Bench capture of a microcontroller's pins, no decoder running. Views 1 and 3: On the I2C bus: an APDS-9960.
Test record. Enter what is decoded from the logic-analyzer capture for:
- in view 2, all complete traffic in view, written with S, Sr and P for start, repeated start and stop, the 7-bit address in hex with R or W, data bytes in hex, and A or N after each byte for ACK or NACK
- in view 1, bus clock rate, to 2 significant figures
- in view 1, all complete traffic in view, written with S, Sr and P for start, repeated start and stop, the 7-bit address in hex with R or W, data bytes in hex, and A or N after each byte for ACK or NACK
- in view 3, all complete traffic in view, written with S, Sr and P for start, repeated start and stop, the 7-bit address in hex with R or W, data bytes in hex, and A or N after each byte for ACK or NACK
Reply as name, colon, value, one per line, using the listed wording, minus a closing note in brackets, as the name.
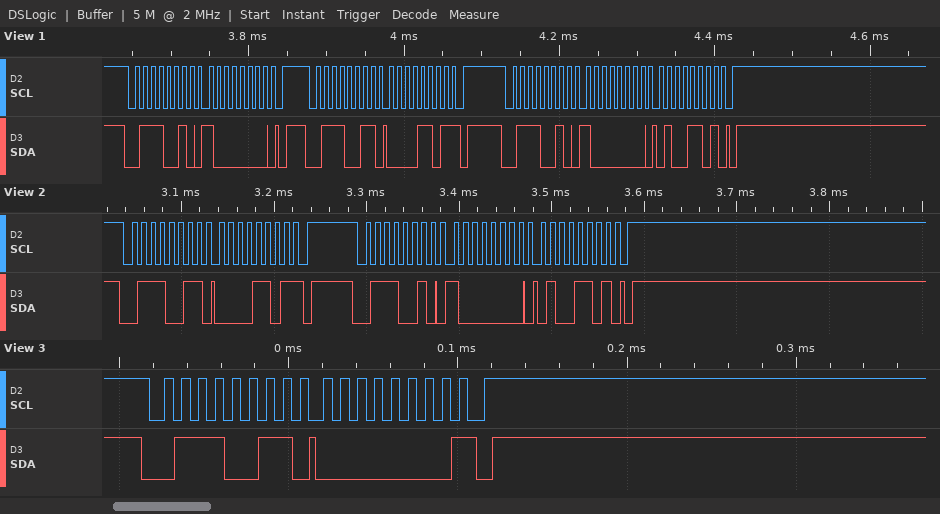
in view 2, all complete traffic in view, written with S, Sr and P for start, repeated start and stop, the 7-bit address in hex with R or W, data bytes in hex, and A or N after each byte for ACK or NACK: S 39R A 0D N P S 39W A 80 A 4D A P
in view 1, bus clock rate, to 2 significant figures: 100 kHz
in view 1, all complete traffic in view, written with S, Sr and P for start, repeated start and stop, the 7-bit address in hex with R or W, data bytes in hex, and A or N after each byte for ACK or NACK: S 39W A 80 A P S 39R A 0D N P S 39W A 80 A 4D A P
in view 3, all complete traffic in view, written with S, Sr and P for start, repeated start and stop, the 7-bit address in hex with R or W, data bytes in hex, and A or N after each byte for ACK or NACK: S 39R A 00 N P
